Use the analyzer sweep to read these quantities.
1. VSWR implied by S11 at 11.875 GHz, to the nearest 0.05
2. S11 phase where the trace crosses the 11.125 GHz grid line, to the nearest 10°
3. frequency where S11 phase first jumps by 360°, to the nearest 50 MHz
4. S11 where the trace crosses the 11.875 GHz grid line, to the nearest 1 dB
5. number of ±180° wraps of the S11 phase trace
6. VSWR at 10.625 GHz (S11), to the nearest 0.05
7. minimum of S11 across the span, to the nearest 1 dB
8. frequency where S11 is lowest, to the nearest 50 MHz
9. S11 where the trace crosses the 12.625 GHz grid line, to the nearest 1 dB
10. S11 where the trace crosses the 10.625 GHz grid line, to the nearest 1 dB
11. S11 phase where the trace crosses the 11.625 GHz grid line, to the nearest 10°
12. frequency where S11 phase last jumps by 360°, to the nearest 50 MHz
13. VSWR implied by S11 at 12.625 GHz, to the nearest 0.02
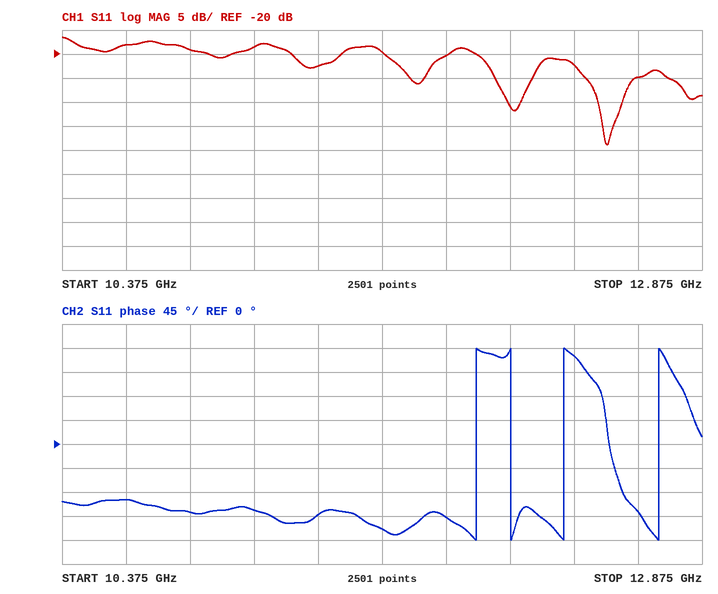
1.20
-120°
12.00 GHz
-20 dB
4
1.30
-39 dB
12.50 GHz
-25 dB
-18 dB
-160°
12.70 GHz
1.12
